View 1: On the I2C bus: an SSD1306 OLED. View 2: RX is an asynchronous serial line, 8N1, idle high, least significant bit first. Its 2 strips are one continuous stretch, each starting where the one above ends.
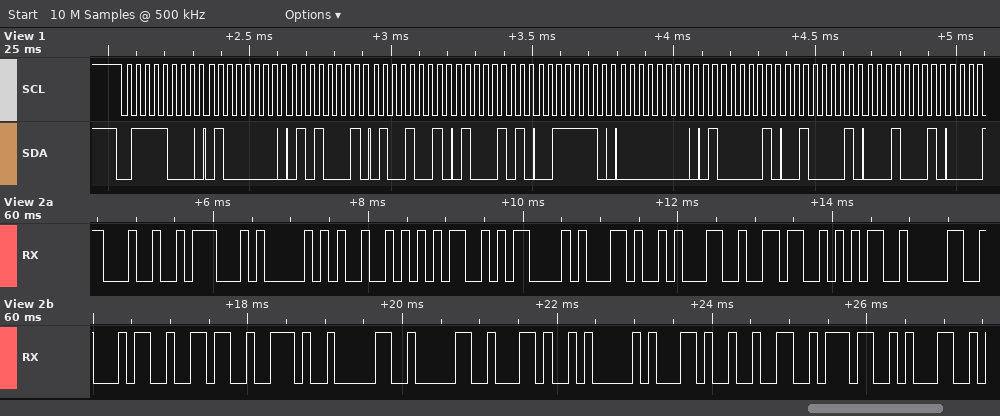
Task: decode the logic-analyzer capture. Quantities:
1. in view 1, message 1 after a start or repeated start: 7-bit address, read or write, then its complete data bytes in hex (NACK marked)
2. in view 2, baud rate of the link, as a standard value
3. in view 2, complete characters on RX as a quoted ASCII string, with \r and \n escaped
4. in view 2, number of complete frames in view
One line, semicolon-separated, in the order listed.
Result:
0x3C write: 40 51 49 45 3E 00 41 21 11; 9600 baud; "$GPRMC,165046.00,A,271"; 22
